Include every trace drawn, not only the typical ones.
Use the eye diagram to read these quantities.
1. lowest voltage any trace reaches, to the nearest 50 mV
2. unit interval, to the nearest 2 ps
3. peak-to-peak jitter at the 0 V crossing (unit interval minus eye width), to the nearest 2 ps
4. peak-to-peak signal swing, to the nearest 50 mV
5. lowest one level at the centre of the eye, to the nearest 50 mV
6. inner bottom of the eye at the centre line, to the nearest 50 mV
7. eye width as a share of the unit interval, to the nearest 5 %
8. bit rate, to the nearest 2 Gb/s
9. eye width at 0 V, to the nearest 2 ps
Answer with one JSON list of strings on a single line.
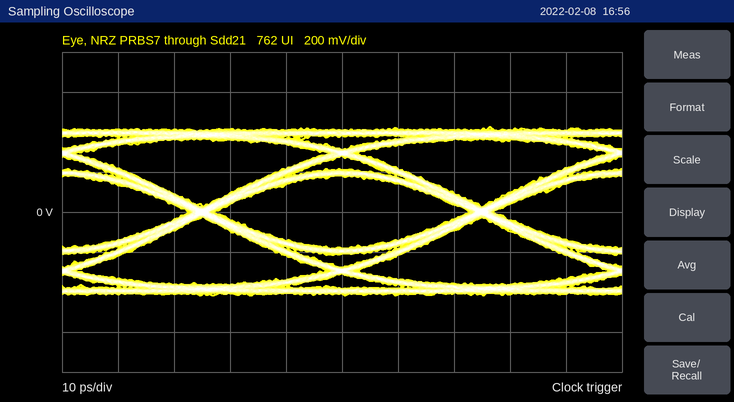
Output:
["-400 mV", "50 ps", "4 ps", "850 mV", "200 mV", "-200 mV", "90 %", "20 Gb/s", "46 ps"]
